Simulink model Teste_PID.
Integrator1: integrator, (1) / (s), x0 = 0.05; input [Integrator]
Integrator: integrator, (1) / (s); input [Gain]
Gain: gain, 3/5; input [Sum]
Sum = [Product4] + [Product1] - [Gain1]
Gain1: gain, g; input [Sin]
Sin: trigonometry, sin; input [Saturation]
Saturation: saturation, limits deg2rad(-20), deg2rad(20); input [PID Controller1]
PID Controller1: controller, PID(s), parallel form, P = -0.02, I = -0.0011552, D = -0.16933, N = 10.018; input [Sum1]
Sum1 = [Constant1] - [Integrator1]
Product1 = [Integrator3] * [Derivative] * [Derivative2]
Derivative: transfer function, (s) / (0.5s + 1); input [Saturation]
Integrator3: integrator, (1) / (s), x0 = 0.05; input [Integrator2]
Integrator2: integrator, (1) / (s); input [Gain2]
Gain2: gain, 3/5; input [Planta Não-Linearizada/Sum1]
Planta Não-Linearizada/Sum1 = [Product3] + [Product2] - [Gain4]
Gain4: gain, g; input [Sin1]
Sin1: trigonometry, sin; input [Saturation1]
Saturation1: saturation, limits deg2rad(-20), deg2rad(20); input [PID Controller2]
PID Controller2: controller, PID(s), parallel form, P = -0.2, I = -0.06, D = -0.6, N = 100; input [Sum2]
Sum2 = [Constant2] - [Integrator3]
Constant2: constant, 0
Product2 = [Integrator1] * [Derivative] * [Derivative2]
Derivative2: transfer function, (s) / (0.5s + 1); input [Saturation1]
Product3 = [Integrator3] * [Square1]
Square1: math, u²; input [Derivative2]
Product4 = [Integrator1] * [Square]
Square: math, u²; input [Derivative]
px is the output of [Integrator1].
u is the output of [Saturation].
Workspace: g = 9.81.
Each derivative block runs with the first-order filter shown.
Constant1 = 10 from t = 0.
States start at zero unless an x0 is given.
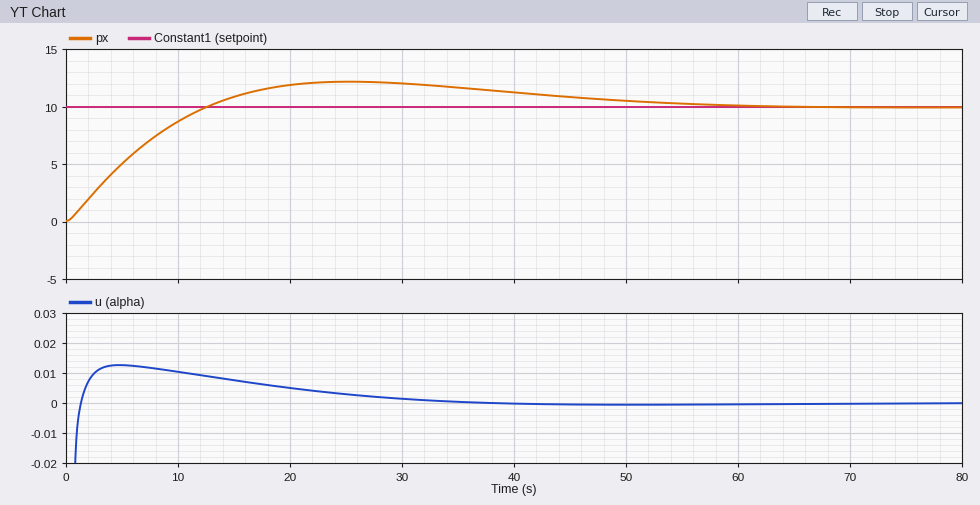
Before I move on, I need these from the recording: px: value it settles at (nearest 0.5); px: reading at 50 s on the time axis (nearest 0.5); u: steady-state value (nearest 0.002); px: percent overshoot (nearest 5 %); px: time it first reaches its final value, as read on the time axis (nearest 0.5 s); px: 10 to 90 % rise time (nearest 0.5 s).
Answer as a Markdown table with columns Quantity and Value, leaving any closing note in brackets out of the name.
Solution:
| Quantity | Value |
|---|---|
| px: value it settles at | 10.0 |
| px: reading at 50 s on the time axis | 10.5 |
| u: steady-state value | 0.000 |
| px: percent overshoot | 20 % |
| px: time it first reaches its final value, as read on the time axis | 12.5 s |
| px: 10 to 90 % rise time | 9.5 s |
